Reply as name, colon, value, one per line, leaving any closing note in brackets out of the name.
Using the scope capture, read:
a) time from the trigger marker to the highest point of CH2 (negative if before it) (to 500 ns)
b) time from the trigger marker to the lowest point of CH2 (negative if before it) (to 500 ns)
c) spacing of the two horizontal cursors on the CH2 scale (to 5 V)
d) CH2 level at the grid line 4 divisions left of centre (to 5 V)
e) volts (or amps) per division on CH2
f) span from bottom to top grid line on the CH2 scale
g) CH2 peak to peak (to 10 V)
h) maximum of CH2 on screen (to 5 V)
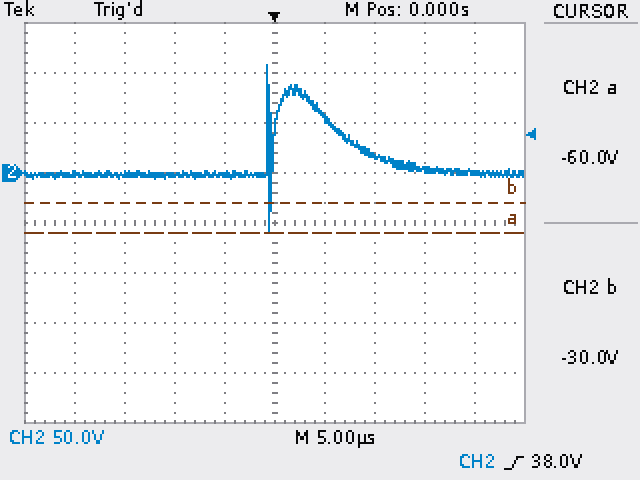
time from the trigger marker to the highest point of CH2 (negative if before it): -500 ns
time from the trigger marker to the lowest point of CH2 (negative if before it): -500 ns
spacing of the two horizontal cursors on the CH2 scale: 30 V
CH2 level at the grid line 4 divisions left of centre: 0 V
volts (or amps) per division on CH2: 50 V
span from bottom to top grid line on the CH2 scale: 400 V
CH2 peak to peak: 170 V
maximum of CH2 on screen: 110 V
